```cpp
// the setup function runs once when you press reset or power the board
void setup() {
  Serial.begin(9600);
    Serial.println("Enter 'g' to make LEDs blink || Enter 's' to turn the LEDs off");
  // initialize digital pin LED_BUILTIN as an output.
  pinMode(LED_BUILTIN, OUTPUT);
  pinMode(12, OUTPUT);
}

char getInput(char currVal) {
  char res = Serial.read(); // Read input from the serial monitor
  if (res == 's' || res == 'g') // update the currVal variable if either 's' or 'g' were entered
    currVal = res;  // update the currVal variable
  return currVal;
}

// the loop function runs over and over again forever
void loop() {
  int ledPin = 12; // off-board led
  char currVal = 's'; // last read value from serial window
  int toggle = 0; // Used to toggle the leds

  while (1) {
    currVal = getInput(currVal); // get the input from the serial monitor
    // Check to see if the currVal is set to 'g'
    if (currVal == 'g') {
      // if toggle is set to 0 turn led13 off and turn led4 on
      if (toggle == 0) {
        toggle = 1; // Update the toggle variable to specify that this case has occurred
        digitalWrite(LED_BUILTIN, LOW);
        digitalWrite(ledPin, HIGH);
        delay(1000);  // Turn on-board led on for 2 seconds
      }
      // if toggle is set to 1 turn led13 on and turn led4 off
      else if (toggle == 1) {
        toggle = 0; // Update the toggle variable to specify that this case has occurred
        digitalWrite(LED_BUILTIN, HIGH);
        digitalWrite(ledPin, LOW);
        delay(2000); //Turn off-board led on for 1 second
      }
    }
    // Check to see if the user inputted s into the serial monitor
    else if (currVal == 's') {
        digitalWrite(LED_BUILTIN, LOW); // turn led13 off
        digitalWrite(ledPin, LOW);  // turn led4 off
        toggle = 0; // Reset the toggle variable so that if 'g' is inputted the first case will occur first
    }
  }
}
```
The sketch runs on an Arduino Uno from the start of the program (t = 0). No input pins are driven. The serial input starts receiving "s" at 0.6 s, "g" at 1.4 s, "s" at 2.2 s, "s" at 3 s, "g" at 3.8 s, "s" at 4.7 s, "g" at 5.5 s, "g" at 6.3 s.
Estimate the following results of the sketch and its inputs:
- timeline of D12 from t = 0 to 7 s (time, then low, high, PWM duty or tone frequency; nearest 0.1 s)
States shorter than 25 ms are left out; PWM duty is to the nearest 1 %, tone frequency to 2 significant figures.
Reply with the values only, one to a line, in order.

0 s low; 1.4 s high; 2.4 s low; 3.8 s high; 4.8 s low; 5.5 s high; 6.5 s low
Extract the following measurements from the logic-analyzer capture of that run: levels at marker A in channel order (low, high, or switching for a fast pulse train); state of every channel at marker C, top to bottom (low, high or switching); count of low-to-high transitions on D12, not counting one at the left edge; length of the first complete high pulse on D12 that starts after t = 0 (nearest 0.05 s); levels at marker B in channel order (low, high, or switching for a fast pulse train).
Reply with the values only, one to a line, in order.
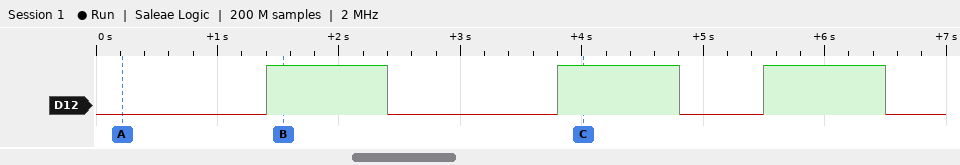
D12 low
D12 high
3
1.00 s
D12 high
